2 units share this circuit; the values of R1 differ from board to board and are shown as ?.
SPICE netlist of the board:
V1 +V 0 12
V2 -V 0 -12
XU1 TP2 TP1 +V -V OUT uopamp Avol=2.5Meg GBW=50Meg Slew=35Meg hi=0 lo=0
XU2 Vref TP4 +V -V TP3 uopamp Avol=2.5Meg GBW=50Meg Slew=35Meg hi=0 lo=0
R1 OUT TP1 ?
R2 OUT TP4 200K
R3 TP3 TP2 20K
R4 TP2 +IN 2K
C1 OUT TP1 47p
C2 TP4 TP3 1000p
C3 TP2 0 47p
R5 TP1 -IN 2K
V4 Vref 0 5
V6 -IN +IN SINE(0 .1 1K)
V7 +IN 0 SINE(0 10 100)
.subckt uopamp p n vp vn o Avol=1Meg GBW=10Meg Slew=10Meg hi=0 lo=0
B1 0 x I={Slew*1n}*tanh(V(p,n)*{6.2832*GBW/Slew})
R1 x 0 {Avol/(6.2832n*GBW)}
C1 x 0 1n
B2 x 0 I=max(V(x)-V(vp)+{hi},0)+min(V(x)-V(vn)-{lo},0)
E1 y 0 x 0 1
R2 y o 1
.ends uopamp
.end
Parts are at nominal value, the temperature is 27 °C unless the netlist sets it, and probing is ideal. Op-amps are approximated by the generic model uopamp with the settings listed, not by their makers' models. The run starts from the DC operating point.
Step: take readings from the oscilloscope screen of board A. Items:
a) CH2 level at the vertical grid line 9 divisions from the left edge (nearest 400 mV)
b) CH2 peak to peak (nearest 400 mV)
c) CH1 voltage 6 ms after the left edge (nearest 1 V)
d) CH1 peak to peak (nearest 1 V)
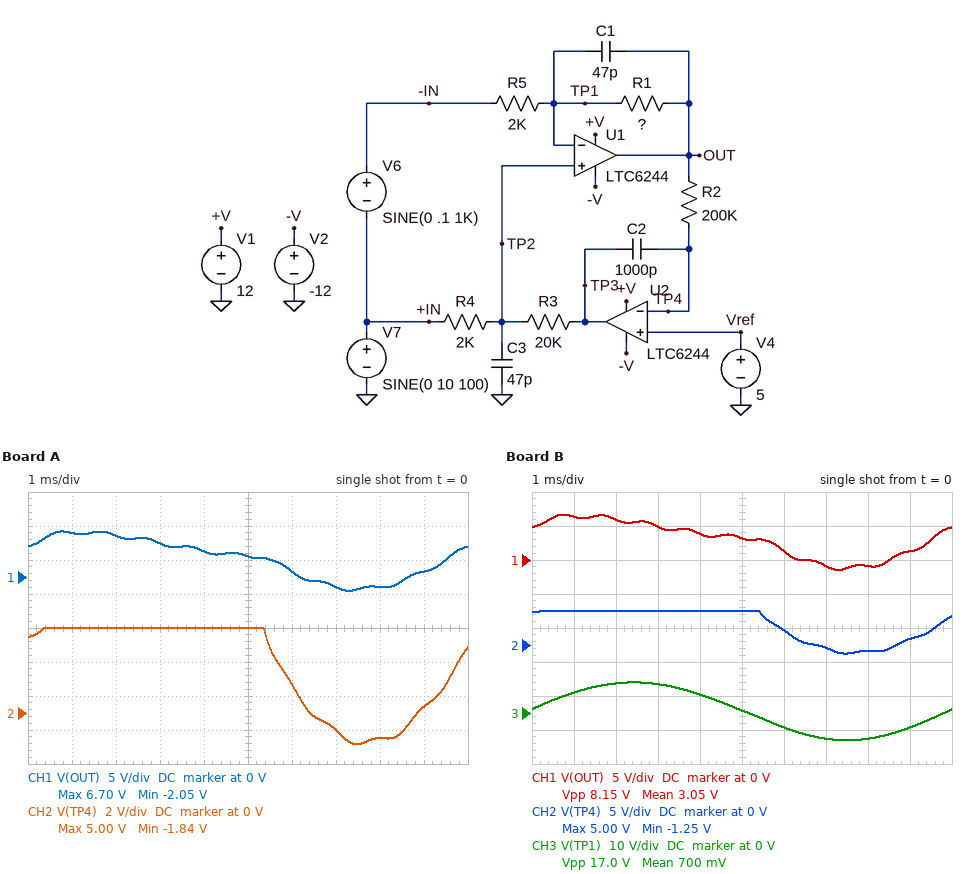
400 mV
6.8 V
1 V
9 V
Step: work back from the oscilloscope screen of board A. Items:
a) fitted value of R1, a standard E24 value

6.2 kΩ
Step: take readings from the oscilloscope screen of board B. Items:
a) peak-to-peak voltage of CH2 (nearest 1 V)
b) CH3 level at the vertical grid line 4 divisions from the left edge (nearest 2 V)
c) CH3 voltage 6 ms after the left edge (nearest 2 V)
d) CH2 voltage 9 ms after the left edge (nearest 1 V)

6 V
6 V
-4 V
1 V
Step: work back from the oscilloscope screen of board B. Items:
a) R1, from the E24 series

6.8 kΩ
